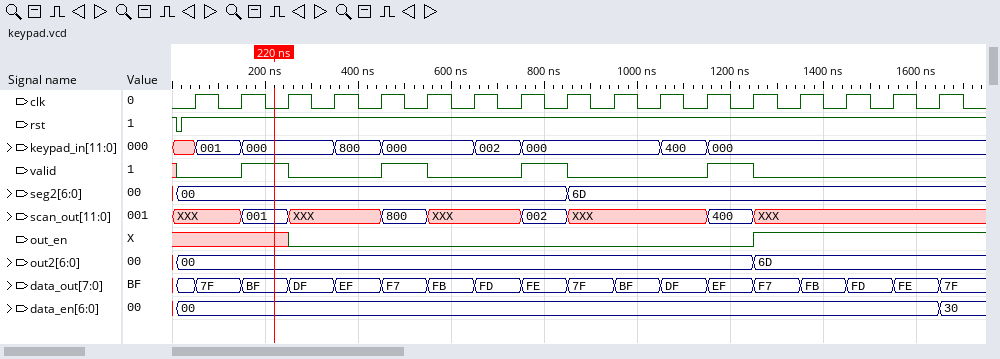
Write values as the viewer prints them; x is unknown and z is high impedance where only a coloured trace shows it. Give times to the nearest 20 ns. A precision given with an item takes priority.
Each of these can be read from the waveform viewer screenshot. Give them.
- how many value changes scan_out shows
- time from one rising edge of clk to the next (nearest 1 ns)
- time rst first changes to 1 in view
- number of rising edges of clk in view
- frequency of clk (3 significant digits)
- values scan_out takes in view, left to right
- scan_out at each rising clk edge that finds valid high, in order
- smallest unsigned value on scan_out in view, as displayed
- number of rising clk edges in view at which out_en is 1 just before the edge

8
100 ns
20 ns
17
10.0 MHz
XXX, 001, XXX, 800, XXX, 002, XXX, 400, XXX
001, 800, 002, 400
001
4
